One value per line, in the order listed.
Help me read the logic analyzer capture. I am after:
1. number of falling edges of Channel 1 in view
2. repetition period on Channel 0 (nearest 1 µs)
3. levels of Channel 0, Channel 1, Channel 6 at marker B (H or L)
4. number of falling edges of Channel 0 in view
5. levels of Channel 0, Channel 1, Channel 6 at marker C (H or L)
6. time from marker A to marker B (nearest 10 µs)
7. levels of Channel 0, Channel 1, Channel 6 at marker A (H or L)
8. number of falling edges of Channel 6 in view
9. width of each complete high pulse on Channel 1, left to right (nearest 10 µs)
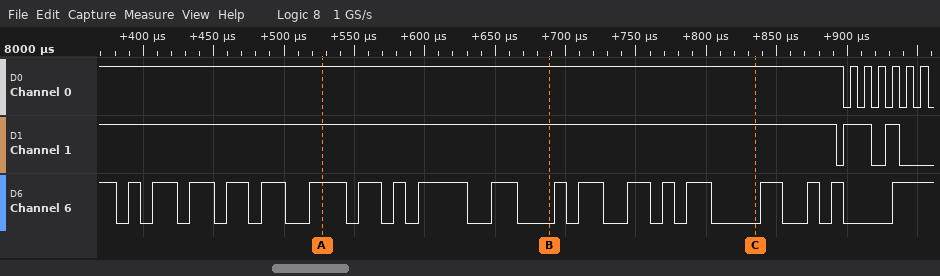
3
10 µs
Channel 0=H, Channel 1=H, Channel 6=L
7
Channel 0=H, Channel 1=H, Channel 6=L
160 µs
Channel 0=H, Channel 1=H, Channel 6=H
19
20 µs, 10 µs
